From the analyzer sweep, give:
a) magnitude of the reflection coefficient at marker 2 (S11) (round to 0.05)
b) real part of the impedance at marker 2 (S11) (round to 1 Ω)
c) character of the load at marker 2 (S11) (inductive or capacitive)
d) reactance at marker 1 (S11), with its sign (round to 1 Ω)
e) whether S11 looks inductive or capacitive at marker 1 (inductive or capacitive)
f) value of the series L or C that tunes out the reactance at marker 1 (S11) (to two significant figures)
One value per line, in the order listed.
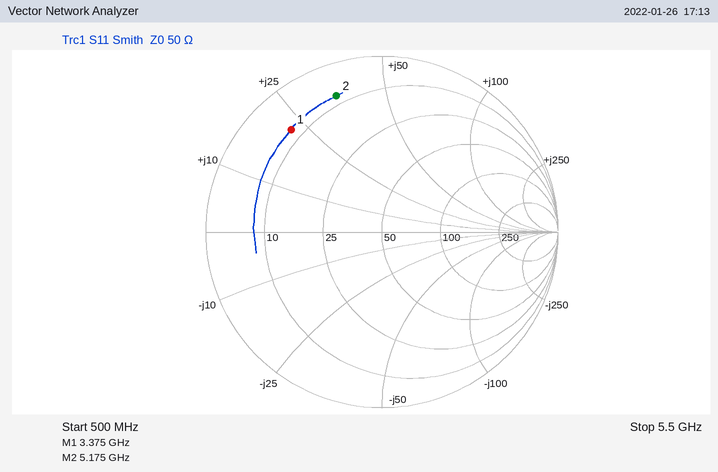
0.80
8 Ω
inductive
+22 Ω
inductive
2.1 pF
